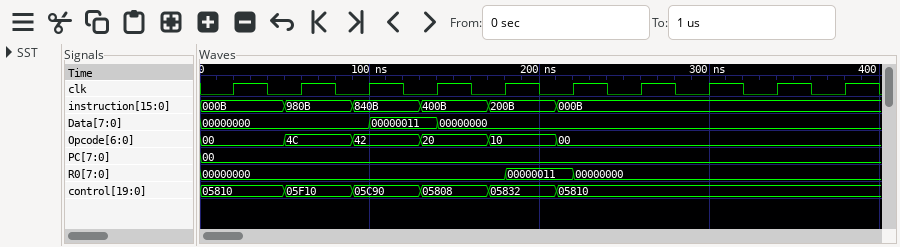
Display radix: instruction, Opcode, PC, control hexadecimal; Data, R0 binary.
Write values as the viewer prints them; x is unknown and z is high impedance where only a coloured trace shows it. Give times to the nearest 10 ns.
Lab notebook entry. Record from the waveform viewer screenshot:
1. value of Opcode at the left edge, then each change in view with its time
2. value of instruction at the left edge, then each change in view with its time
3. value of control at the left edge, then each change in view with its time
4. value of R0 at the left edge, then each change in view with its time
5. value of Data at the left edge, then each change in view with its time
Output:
00, 4C at 50 ns, 42 at 90 ns, 20 at 130 ns, 10 at 170 ns, 00 at 210 ns
000B, 980B at 50 ns, 840B at 90 ns, 400B at 130 ns, 200B at 170 ns, 000B at 210 ns
05810, 05F10 at 50 ns, 05C90 at 90 ns, 05808 at 130 ns, 05832 at 170 ns, 05810 at 210 ns
00000000, 00000011 at 180 ns, 00000000 at 220 ns
00000000, 00000011 at 100 ns, 00000000 at 140 ns
